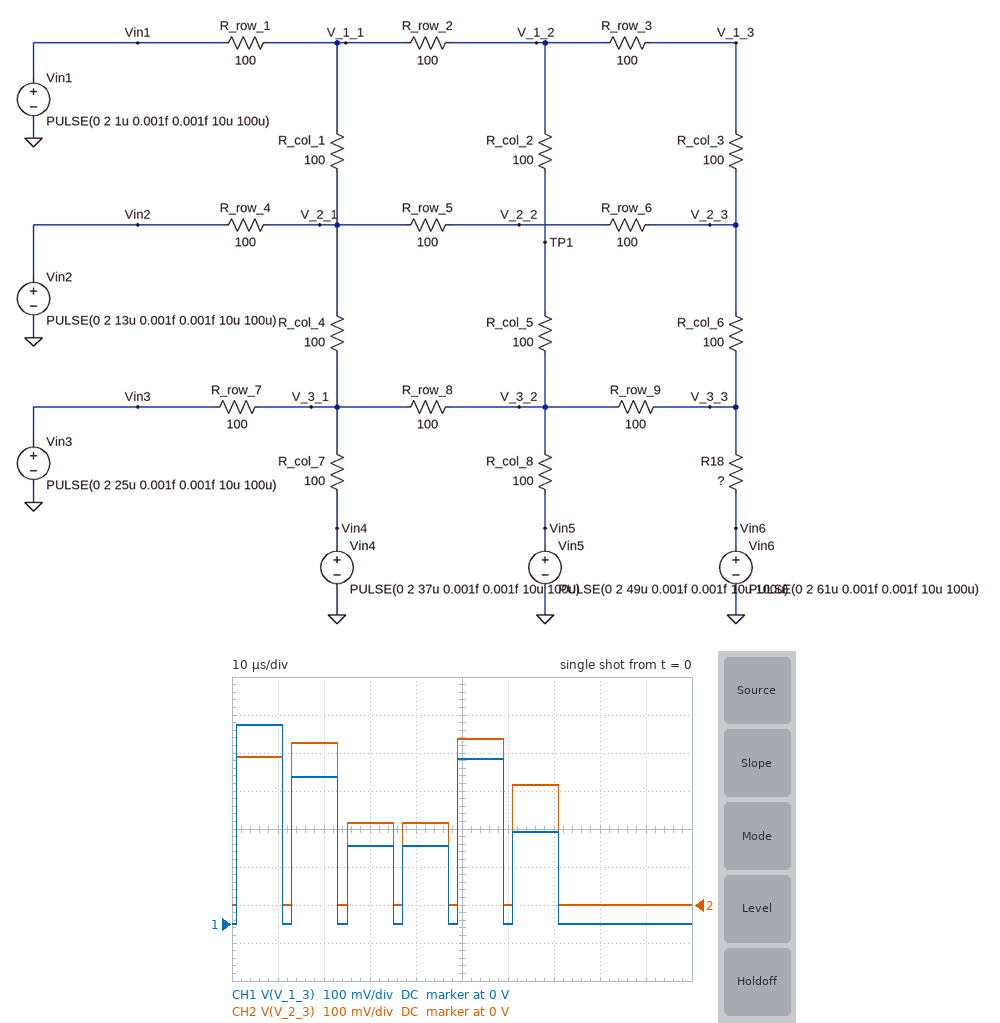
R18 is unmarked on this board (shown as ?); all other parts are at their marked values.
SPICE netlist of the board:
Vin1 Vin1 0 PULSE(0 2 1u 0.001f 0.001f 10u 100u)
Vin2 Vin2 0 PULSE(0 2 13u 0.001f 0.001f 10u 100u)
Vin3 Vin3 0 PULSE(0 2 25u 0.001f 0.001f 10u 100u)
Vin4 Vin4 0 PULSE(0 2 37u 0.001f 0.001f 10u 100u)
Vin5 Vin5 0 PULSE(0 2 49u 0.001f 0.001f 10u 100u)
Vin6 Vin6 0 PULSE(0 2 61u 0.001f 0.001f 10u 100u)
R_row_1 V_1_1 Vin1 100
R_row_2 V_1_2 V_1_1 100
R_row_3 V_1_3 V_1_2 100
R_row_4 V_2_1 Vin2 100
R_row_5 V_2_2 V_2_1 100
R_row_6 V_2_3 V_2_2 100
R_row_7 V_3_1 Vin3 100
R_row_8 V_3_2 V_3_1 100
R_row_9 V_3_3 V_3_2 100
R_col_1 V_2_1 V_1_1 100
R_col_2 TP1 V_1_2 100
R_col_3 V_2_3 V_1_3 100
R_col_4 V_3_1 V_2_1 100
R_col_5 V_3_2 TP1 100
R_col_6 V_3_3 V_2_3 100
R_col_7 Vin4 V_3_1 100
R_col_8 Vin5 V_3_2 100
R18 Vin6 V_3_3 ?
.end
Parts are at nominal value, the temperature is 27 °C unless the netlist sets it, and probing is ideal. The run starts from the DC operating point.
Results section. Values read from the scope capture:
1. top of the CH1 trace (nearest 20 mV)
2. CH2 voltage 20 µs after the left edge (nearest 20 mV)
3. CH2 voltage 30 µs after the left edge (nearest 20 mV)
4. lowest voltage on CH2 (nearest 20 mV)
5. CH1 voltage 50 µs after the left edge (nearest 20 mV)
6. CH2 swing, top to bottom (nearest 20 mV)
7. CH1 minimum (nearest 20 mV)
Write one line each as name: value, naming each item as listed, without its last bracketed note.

top of the CH1 trace: 520 mV
CH2 voltage 20 µs after the left edge: 420 mV
CH2 voltage 30 µs after the left edge: 220 mV
lowest voltage on CH2: 0 V
CH1 voltage 50 µs after the left edge: 440 mV
CH2 swing, top to bottom: 440 mV
CH1 minimum: 0 V
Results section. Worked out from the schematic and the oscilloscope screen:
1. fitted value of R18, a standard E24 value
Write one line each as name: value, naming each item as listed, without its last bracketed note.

fitted value of R18, a standard E24 value: 300 Ω
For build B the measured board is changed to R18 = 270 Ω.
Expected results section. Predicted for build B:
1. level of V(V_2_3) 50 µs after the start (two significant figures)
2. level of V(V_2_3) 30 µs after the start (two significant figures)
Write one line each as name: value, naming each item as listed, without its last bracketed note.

level of V(V_2_3) 50 µs after the start: 430 mV
level of V(V_2_3) 30 µs after the start: 210 mV
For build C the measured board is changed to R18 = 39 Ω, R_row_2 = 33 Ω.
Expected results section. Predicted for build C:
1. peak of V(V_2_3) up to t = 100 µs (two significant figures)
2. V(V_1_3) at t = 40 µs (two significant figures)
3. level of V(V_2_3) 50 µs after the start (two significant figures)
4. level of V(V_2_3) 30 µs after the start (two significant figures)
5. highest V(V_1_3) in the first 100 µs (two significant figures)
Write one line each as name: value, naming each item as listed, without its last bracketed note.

peak of V(V_2_3) up to t = 100 µs: 880 mV
V(V_1_3) at t = 40 µs: 140 mV
level of V(V_2_3) 50 µs after the start: 200 mV
level of V(V_2_3) 30 µs after the start: 130 mV
highest V(V_1_3) in the first 100 µs: 630 mV
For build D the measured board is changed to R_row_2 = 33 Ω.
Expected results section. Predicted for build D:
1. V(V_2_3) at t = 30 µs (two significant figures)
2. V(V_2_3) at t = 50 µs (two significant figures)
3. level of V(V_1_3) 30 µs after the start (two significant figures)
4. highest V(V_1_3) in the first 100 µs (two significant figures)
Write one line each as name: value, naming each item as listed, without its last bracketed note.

V(V_2_3) at t = 30 µs: 210 mV
V(V_2_3) at t = 50 µs: 400 mV
level of V(V_1_3) 30 µs after the start: 190 mV
highest V(V_1_3) in the first 100 µs: 630 mV
